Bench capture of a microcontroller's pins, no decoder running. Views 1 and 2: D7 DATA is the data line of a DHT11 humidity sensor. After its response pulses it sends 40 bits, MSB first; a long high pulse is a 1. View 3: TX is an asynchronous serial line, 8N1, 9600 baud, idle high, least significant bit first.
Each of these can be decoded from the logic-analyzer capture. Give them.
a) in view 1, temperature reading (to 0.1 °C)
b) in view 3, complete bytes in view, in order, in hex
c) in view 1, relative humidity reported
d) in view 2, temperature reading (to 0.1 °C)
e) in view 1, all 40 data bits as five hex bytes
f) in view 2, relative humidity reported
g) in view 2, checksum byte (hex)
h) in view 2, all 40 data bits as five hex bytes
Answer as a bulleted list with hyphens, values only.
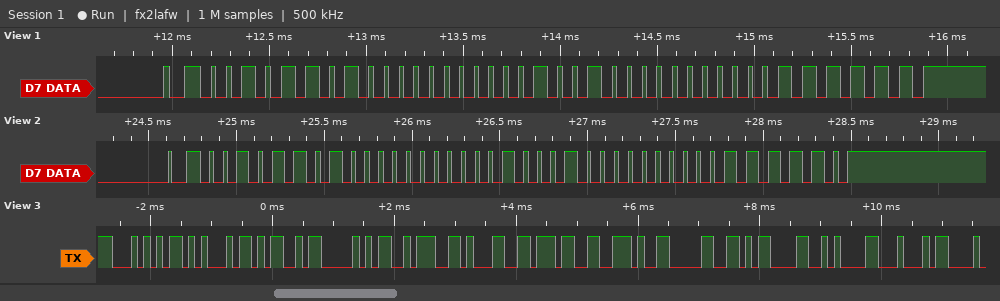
- 18.0 °C
- 54 45 4D 50 3A 31 37 2E 30 0D 0A 44
- 45 %
- 17.0 °C
- 2D 00 12 00 3F
- 45 %
- 0x3E
- 2D 00 11 00 3E
